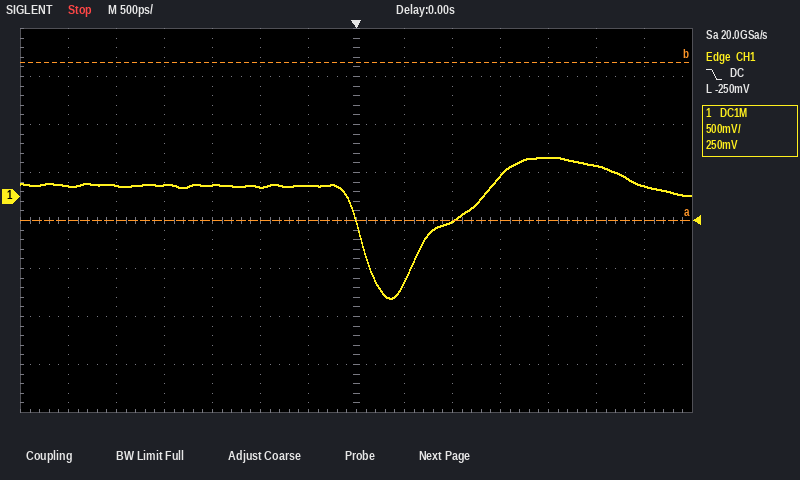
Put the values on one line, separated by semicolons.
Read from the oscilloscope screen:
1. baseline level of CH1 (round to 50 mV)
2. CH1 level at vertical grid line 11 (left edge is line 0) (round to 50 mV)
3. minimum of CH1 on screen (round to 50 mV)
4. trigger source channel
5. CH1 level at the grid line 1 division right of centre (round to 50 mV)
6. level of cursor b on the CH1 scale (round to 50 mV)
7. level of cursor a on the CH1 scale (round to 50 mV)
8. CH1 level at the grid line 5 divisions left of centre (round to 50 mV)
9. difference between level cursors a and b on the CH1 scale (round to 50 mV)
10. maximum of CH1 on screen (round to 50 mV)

100 mV; 400 mV; -1.05 V; CH1; -900 mV; 1.40 V; -250 mV; 100 mV; 1.65 V; 400 mV
